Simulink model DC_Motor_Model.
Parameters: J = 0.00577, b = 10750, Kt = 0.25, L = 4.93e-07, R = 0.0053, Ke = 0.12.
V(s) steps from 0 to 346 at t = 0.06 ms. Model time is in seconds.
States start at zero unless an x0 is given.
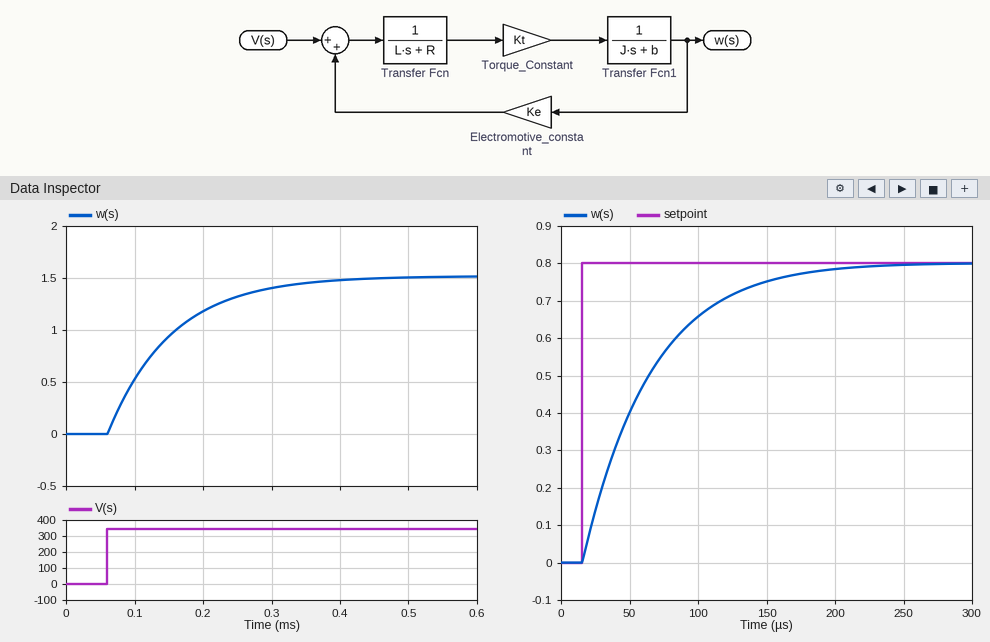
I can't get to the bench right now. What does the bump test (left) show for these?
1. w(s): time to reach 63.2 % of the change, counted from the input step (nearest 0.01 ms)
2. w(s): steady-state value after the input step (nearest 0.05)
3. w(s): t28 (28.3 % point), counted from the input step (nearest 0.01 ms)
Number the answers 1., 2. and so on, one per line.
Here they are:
1. 0.09 ms
2. 1.50
3. 0.03 ms
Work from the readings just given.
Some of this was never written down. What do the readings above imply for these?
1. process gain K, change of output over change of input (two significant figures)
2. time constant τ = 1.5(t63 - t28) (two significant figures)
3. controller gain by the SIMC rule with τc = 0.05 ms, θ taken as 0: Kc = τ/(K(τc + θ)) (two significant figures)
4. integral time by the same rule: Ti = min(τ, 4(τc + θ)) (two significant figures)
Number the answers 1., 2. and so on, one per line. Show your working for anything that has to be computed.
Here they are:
1. (1.5 - 0) / 346 = 0.0043
2. 1.5 × (0.09 - 0.03) = 0.090 ms
3. 0.09 / (0.0043 × (0.05 + 0)) = 420
4. min(0.09, 4 × (0.05 + 0)) = 0.090 ms
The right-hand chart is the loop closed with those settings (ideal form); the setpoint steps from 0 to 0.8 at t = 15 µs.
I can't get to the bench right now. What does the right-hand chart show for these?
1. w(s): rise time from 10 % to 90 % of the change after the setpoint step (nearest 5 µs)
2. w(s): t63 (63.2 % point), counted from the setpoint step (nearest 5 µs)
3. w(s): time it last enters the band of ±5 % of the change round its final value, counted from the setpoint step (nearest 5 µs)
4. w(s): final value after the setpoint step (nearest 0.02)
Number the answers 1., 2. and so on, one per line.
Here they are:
1. 105 µs
2. 50 µs
3. 145 µs
4. 0.80
